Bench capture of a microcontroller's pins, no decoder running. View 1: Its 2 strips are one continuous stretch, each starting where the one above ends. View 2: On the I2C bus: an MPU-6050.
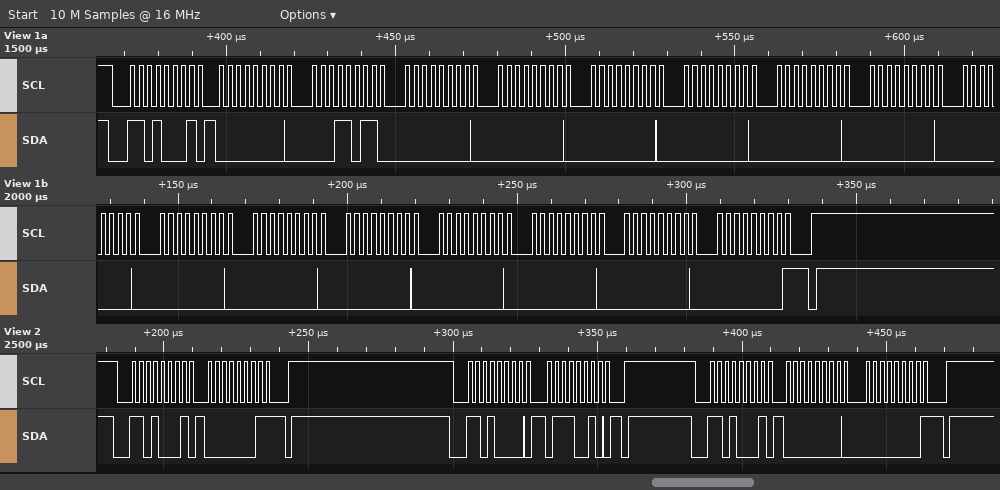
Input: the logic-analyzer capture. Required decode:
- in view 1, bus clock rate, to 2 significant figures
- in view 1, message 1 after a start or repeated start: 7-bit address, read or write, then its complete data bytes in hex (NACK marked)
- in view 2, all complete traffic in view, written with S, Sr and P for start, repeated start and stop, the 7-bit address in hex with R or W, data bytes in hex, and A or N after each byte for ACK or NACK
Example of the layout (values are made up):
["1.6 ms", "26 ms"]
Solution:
["400 kHz", "0x68 read: 00 1B 00 00 00 00 00 00 00 00 00 00 00 00 00 00 NACK", "S 68R A 01 N P S 68W A 72 A P S 68R A 00 A 00 N P"]
